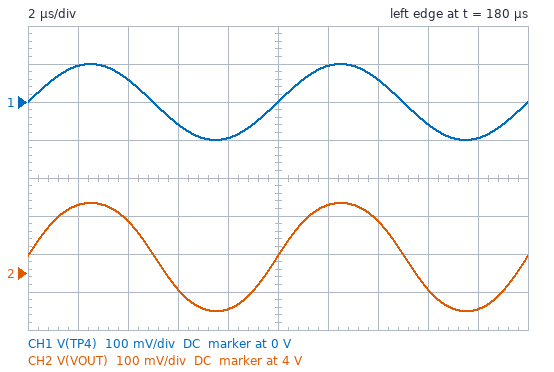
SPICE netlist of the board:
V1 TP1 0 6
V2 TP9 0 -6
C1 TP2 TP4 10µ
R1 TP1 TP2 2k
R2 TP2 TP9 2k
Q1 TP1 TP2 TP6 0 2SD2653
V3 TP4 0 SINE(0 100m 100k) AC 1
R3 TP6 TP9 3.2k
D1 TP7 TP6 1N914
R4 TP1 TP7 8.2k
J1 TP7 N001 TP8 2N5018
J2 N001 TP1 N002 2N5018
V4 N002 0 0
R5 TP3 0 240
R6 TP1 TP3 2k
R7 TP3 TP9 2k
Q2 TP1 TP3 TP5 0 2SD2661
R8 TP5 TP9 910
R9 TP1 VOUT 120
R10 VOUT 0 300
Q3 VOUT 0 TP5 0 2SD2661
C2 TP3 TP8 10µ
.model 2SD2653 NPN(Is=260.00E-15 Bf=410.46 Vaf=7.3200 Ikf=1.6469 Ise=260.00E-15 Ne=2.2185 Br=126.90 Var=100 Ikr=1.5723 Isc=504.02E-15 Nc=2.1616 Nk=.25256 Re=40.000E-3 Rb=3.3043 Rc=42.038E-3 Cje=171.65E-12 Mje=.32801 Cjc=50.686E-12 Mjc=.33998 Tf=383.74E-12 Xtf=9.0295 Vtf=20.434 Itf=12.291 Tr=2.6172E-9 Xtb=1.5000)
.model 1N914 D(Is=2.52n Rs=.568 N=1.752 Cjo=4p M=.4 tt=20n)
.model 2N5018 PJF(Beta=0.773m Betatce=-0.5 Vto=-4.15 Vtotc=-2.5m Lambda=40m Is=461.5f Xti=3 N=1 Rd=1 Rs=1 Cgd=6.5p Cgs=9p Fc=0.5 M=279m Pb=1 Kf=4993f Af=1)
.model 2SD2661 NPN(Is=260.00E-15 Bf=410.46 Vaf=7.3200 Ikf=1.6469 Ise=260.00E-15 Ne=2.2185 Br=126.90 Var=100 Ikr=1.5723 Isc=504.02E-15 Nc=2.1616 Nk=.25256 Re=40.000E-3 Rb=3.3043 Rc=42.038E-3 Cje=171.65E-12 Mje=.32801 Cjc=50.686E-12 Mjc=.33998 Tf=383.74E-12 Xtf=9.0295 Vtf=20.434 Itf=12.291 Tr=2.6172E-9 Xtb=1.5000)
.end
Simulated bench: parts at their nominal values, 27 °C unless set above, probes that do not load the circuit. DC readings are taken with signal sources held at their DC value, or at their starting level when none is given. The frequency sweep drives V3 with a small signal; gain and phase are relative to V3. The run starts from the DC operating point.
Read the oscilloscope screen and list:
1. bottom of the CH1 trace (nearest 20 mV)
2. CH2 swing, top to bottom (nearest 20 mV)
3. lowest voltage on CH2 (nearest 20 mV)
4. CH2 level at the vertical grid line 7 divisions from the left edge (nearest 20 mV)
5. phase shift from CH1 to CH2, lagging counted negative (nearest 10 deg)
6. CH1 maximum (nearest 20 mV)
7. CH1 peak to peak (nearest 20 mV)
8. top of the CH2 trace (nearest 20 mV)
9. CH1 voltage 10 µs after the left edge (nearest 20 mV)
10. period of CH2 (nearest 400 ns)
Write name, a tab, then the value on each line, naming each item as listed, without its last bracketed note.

bottom of the CH1 trace	-100 mV
CH2 swing, top to bottom	280 mV
lowest voltage on CH2	3.90 V
CH2 level at the vertical grid line 7 divisions from the left edge	4.14 V
phase shift from CH1 to CH2, lagging counted negative	0 deg
CH1 maximum	100 mV
CH1 peak to peak	200 mV
top of the CH2 trace	4.18 V
CH1 voltage 10 µs after the left edge	0 V
period of CH2	10.0 µs
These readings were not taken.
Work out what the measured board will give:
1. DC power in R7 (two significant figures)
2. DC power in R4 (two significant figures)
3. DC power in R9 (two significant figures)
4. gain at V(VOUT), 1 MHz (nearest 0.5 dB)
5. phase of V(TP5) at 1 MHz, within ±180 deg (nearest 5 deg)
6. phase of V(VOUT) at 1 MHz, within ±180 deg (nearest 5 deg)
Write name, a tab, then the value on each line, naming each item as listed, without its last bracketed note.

DC power in R7	18 mW
DC power in R4	4.4 mW
DC power in R9	32 mW
gain at V(VOUT), 1 MHz	4.0 dB
phase of V(TP5) at 1 MHz, within ±180 deg	-5 deg
phase of V(VOUT) at 1 MHz, within ±180 deg	-10 deg
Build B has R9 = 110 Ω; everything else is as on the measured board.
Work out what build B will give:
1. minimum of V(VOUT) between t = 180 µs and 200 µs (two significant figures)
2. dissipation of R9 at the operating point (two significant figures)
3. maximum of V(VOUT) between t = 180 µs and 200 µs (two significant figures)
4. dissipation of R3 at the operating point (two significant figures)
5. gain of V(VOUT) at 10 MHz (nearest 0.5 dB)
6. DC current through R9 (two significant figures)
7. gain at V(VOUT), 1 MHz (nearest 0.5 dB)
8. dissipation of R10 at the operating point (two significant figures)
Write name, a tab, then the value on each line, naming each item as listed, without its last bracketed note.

minimum of V(VOUT) between t = 180 µs and 200 µs	4.0 V
dissipation of R9 at the operating point	31 mW
maximum of V(VOUT) between t = 180 µs and 200 µs	4.3 V
dissipation of R3 at the operating point	9.3 mW
gain of V(VOUT) at 10 MHz	-0.5 dB
DC current through R9	17 mA
gain at V(VOUT), 1 MHz	3.5 dB
dissipation of R10 at the operating point	58 mW
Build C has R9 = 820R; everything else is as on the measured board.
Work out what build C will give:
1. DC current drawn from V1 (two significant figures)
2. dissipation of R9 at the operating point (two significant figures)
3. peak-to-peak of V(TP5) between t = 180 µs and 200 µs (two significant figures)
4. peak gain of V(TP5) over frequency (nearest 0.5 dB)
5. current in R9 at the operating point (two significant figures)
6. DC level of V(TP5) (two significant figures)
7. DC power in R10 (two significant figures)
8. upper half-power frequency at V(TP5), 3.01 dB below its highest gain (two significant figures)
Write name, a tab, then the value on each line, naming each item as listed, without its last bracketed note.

DC current drawn from V1	17 mA
dissipation of R9 at the operating point	29 mW
peak-to-peak of V(TP5) between t = 180 µs and 200 µs	40 mV
peak gain of V(TP5) over frequency	-14.0 dB
current in R9 at the operating point	6.0 mA
DC level of V(TP5)	-590 mV
DC power in R10	4.0 mW
upper half-power frequency at V(TP5), 3.01 dB below its highest gain	10 MHz
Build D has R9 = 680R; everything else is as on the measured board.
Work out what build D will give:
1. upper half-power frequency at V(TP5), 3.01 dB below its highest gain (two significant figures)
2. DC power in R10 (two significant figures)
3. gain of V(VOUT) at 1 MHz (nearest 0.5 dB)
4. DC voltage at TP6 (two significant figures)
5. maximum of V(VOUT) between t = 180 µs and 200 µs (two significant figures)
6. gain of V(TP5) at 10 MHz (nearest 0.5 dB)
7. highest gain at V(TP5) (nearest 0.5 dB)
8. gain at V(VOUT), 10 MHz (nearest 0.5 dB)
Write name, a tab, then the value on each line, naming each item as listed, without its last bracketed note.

upper half-power frequency at V(TP5), 3.01 dB below its highest gain	9.8 MHz
DC power in R10	6.0 mW
gain of V(VOUT) at 1 MHz	11.0 dB
DC voltage at TP6	-560 mV
maximum of V(VOUT) between t = 180 µs and 200 µs	1.6 V
gain of V(TP5) at 10 MHz	-17.0 dB
highest gain at V(TP5)	-14.0 dB
gain at V(VOUT), 10 MHz	7.0 dB
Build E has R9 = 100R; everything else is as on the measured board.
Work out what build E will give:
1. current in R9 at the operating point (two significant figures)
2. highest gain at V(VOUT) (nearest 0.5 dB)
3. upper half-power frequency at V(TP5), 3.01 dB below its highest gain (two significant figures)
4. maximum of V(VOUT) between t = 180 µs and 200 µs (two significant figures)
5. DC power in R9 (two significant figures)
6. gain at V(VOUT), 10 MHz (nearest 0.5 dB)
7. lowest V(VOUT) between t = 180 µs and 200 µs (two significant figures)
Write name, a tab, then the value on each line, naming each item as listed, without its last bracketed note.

current in R9 at the operating point	17 mA
highest gain at V(VOUT)	3.0 dB
upper half-power frequency at V(TP5), 3.01 dB below its highest gain	8.0 MHz
maximum of V(VOUT) between t = 180 µs and 200 µs	4.4 V
DC power in R9	29 mW
gain at V(VOUT), 10 MHz	-1.0 dB
lowest V(VOUT) between t = 180 µs and 200 µs	4.2 V
